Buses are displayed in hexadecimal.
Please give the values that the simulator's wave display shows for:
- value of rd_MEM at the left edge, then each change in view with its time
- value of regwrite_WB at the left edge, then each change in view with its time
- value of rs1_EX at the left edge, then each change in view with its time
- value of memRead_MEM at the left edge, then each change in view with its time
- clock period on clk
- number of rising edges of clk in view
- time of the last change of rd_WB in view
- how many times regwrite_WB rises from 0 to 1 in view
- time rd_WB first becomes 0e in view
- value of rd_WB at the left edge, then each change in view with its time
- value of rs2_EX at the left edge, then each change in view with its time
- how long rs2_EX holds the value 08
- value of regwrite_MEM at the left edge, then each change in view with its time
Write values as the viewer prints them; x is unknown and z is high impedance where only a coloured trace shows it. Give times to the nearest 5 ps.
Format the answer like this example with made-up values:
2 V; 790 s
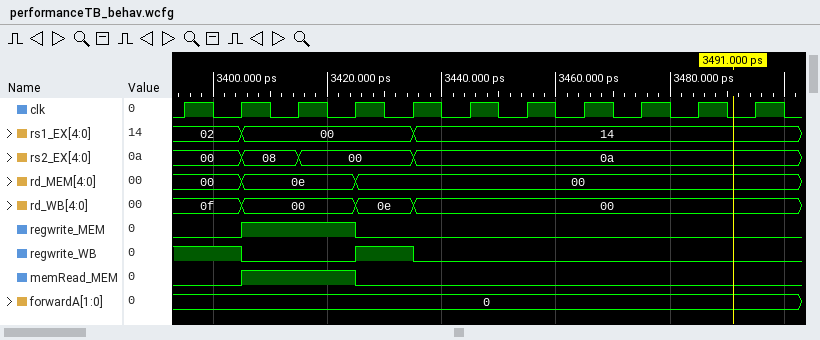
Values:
00, 0e at 3405 ps, 00 at 3425 ps; 1, 0 at 3405 ps, 1 at 3425 ps, 0 at 3435 ps; 02, 00 at 3405 ps, 14 at 3435 ps; 0, 1 at 3405 ps, 0 at 3425 ps; 10 ps; 11; 3435 ps; 1; 3425 ps; 0f, 00 at 3405 ps, 0e at 3425 ps, 00 at 3435 ps; 00, 08 at 3405 ps, 00 at 3415 ps, 0a at 3435 ps; 10 ps; 0, 1 at 3405 ps, 0 at 3425 ps
